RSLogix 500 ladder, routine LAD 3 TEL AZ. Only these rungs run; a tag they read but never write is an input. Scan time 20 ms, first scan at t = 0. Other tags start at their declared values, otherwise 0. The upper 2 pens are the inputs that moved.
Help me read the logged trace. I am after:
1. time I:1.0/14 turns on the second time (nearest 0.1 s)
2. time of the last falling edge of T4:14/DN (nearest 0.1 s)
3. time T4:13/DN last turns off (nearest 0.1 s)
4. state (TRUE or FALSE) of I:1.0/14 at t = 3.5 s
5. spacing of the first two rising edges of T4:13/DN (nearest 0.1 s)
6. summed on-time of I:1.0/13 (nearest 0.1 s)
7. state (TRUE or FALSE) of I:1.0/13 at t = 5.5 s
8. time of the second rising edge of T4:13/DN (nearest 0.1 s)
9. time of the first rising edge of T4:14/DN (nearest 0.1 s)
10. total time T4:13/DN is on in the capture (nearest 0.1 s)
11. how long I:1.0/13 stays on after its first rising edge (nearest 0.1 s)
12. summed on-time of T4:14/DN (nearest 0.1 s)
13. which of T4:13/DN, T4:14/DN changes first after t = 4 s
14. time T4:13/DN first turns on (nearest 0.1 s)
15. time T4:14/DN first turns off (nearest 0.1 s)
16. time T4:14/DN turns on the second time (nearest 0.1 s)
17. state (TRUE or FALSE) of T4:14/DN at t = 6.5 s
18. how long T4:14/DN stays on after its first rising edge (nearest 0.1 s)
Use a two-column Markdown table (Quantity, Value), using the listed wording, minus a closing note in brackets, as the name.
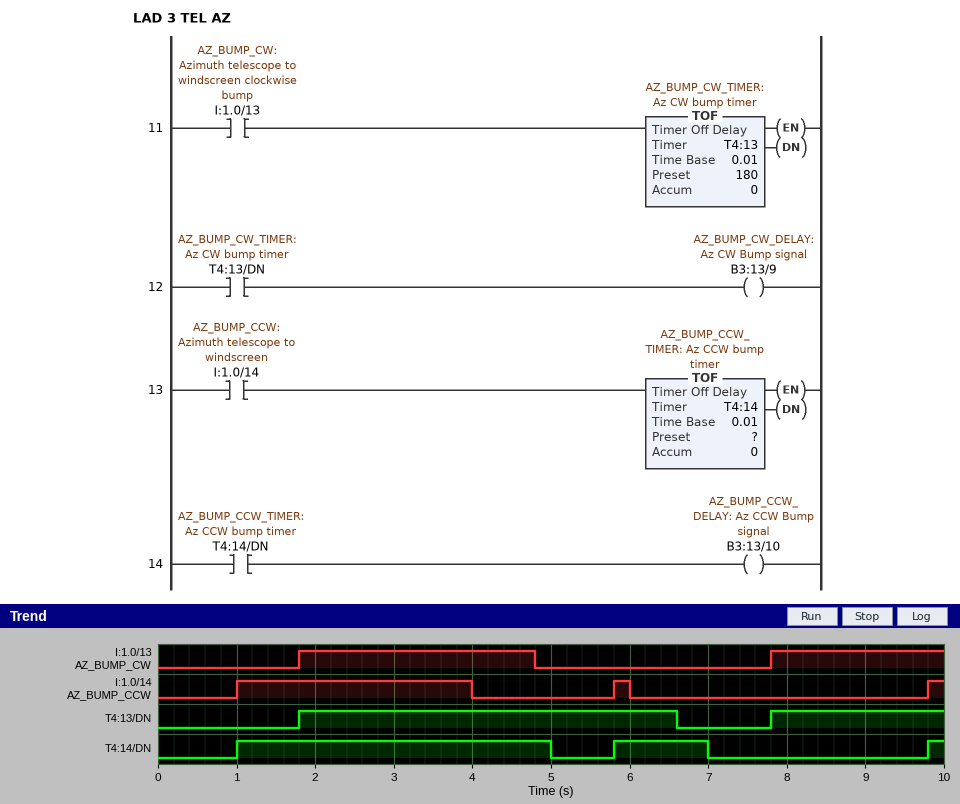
| Quantity | Value |
|---|---|
| time I:1.0/14 turns on the second time | 5.8 s |
| time of the last falling edge of T4:14/DN | 7.0 s |
| time T4:13/DN last turns off | 6.6 s |
| state (TRUE or FALSE) of I:1.0/14 at t = 3.5 s | TRUE |
| spacing of the first two rising edges of T4:13/DN | 6.0 s |
| summed on-time of I:1.0/13 | 5.2 s |
| state (TRUE or FALSE) of I:1.0/13 at t = 5.5 s | FALSE |
| time of the second rising edge of T4:13/DN | 7.8 s |
| time of the first rising edge of T4:14/DN | 1.0 s |
| total time T4:13/DN is on in the capture | 7.0 s |
| how long I:1.0/13 stays on after its first rising edge | 3.0 s |
| summed on-time of T4:14/DN | 5.4 s |
| which of T4:13/DN, T4:14/DN changes first after t = 4 s | T4:14/DN |
| time T4:13/DN first turns on | 1.8 s |
| time T4:14/DN first turns off | 5.0 s |
| time T4:14/DN turns on the second time | 5.8 s |
| state (TRUE or FALSE) of T4:14/DN at t = 6.5 s | TRUE |
| how long T4:14/DN stays on after its first rising edge | 4.0 s |
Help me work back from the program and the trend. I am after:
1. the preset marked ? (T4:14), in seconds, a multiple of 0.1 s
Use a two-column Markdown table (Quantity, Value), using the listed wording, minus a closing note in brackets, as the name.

| Quantity | Value |
|---|---|
| the preset marked ? (T4:14), in seconds, a multiple of 0.1 s | 1.0 s |
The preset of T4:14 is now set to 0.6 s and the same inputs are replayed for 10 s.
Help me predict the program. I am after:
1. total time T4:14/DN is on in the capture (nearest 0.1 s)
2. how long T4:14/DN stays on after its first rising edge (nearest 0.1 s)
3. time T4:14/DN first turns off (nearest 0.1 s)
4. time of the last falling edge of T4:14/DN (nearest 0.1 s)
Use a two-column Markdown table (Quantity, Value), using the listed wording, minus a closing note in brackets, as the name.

| Quantity | Value |
|---|---|
| total time T4:14/DN is on in the capture | 4.6 s |
| how long T4:14/DN stays on after its first rising edge | 3.6 s |
| time T4:14/DN first turns off | 4.6 s |
| time of the last falling edge of T4:14/DN | 6.6 s |
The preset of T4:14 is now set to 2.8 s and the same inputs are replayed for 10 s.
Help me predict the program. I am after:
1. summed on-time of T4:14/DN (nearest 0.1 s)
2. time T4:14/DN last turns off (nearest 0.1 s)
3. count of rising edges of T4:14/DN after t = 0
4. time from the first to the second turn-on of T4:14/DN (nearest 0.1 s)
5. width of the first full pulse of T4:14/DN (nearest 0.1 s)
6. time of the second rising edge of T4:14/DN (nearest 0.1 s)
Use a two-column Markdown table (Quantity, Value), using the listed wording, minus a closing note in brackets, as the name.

| Quantity | Value |
|---|---|
| summed on-time of T4:14/DN | 8.0 s |
| time T4:14/DN last turns off | 8.8 s |
| count of rising edges of T4:14/DN after t = 0 | 2 |
| time from the first to the second turn-on of T4:14/DN | 8.8 s |
| width of the first full pulse of T4:14/DN | 7.8 s |
| time of the second rising edge of T4:14/DN | 9.8 s |
